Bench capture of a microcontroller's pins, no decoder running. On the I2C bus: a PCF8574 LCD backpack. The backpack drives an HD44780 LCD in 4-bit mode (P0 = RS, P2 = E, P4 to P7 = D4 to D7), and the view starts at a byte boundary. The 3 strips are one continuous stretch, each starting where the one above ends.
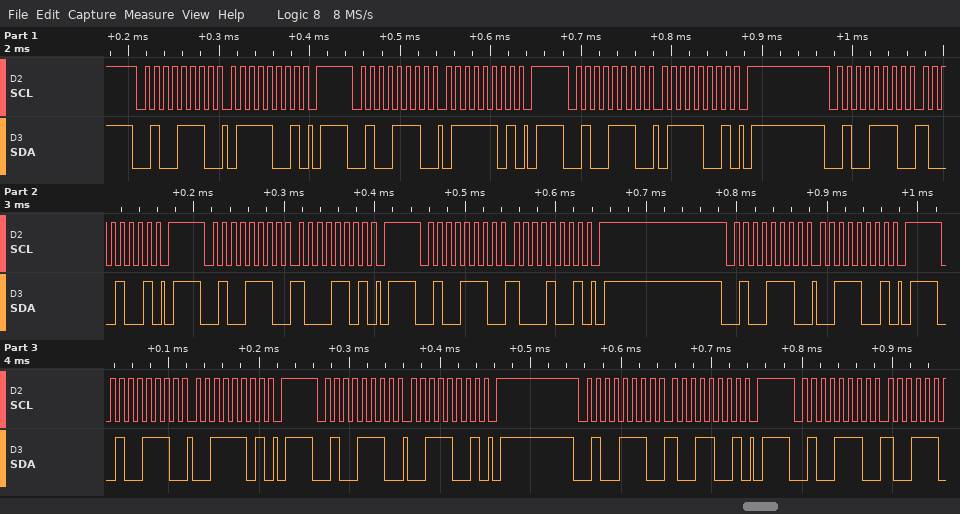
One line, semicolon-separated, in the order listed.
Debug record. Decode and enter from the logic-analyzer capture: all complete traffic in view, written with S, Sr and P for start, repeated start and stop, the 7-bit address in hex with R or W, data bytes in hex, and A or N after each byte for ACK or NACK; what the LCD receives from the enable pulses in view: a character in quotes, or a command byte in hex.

S 27W A 79 A P S 27W A 7D A P S 27W A 79 A P S 27W A 89 A P S 27W A 8D A P S 27W A 89 A P S 27W A 39 A P S 27W A 3D A P S 27W A 39 A P S 27W A 99 A P S 27W A; 'x'
